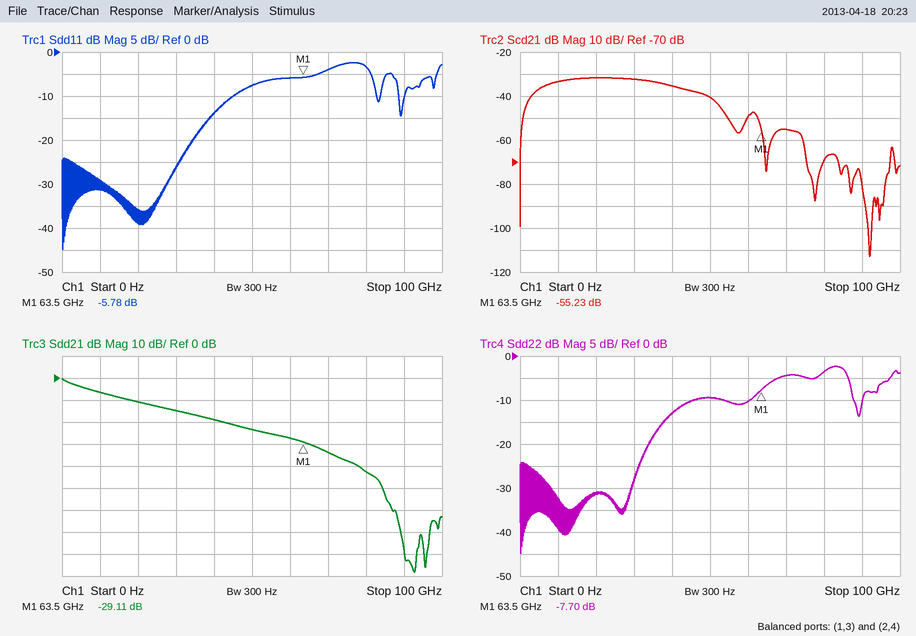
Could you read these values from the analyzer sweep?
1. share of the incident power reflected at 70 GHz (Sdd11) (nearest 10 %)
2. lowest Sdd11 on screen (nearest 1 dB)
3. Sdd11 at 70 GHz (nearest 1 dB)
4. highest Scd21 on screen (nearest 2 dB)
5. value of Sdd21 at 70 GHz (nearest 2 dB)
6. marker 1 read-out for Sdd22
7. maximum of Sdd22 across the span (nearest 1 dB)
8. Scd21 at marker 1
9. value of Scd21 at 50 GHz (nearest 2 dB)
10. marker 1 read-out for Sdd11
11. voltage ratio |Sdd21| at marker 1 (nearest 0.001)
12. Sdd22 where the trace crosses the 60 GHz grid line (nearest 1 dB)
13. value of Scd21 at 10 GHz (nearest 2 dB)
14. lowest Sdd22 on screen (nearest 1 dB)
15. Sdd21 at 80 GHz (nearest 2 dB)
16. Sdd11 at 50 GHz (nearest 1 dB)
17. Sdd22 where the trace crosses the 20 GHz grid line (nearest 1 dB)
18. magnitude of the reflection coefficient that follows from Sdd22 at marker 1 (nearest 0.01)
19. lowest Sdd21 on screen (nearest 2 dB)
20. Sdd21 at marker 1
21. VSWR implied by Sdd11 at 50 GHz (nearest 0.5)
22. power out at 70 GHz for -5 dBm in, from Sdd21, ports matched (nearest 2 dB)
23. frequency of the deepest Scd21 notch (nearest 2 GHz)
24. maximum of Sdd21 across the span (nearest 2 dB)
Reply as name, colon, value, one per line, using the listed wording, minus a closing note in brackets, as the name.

share of the incident power reflected at 70 GHz (Sdd11): 40 %
lowest Sdd11 on screen: -45 dB
Sdd11 at 70 GHz: -4 dB
highest Scd21 on screen: -32 dB
value of Sdd21 at 70 GHz: -34 dB
marker 1 read-out for Sdd22: -7.70 dB
maximum of Sdd22 across the span: -2 dB
Scd21 at marker 1: -55.23 dB
value of Scd21 at 50 GHz: -40 dB
marker 1 read-out for Sdd11: -5.78 dB
voltage ratio |Sdd21| at marker 1: 0.035
Sdd22 where the trace crosses the 60 GHz grid line: -10 dB
value of Scd21 at 10 GHz: -34 dB
lowest Sdd22 on screen: -45 dB
Sdd21 at 80 GHz: -42 dB
Sdd11 at 50 GHz: -8 dB
Sdd22 where the trace crosses the 20 GHz grid line: -31 dB
magnitude of the reflection coefficient that follows from Sdd22 at marker 1: 0.41
lowest Sdd21 on screen: -88 dB
Sdd21 at marker 1: -29.11 dB
VSWR implied by Sdd11 at 50 GHz: 2.5
power out at 70 GHz for -5 dBm in, from Sdd21, ports matched: -38 dBm
frequency of the deepest Scd21 notch: 92 GHz
maximum of Sdd21 across the span: 0 dB
